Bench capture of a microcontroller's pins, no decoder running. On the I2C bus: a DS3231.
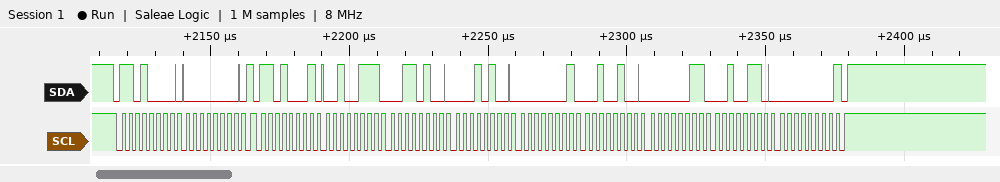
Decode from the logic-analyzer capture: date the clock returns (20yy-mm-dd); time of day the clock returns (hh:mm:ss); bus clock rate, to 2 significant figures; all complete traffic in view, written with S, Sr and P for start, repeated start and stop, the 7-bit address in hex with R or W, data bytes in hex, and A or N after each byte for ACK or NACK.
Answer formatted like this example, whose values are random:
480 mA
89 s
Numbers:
2026-03-24
14:34:27
400 kHz
S 68W A 00 A Sr 68R A 27 A 34 A 14 A 01 A 24 A 03 A 26 A 00 N P
